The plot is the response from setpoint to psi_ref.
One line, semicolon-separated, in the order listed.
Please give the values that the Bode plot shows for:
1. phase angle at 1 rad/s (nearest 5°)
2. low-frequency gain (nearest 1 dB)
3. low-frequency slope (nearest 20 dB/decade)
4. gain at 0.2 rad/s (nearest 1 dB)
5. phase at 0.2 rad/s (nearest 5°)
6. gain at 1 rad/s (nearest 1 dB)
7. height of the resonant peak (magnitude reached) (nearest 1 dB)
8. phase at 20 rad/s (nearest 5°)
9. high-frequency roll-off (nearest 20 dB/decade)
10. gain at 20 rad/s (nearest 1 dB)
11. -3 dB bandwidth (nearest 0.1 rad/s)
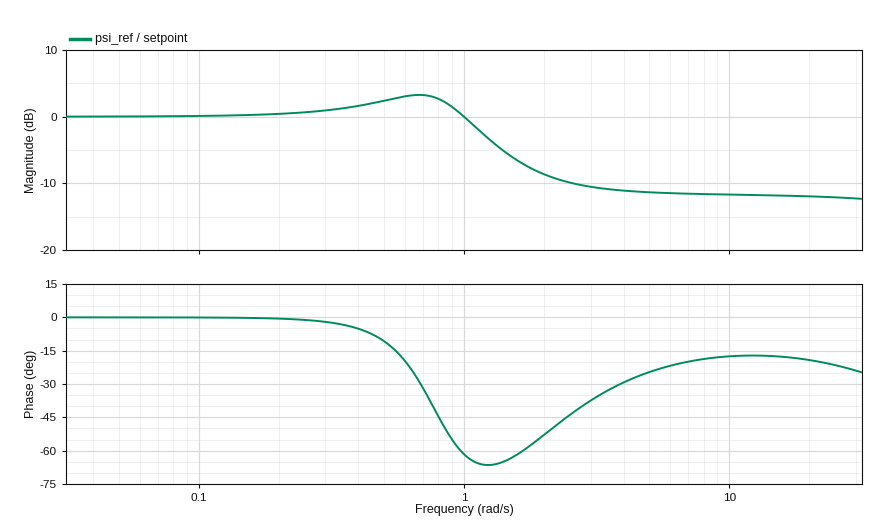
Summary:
-60°; 0 dB; 0 dB/decade; 0 dB; 0°; 0 dB; 3 dB; -20°; 0 dB/decade; -12 dB; 1.2 rad/s
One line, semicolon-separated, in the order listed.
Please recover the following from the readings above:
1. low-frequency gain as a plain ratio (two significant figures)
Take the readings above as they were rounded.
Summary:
1.0
